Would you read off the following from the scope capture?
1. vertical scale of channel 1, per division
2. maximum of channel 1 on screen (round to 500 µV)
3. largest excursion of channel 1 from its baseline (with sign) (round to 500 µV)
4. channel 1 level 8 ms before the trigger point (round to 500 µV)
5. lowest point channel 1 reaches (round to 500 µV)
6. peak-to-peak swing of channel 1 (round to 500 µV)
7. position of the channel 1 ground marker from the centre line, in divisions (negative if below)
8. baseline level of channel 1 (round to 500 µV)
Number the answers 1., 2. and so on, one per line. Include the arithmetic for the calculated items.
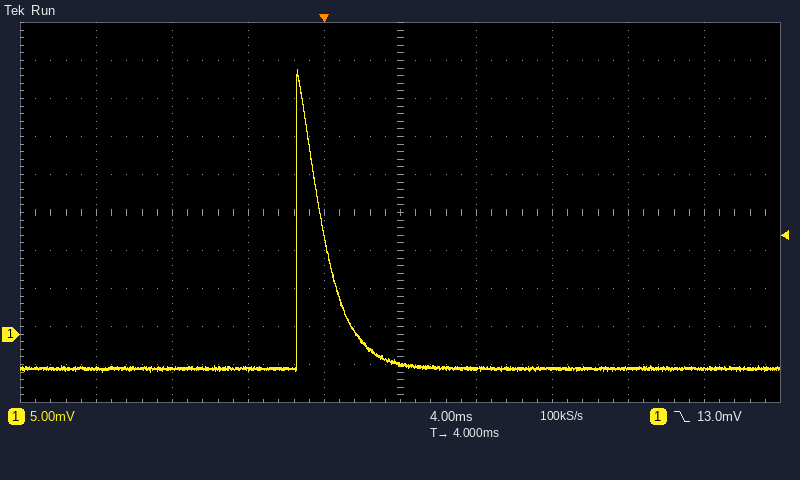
1. 5 mV
2. 35.0 mV
3. 35.0 mV − (-4.5 mV) = +39.5 mV
4. -4.5 mV
5. -5.0 mV
6. 35.0 mV − (-5.0 mV) = 40.0 mV
7. -3.2 div
8. -4.5 mV
